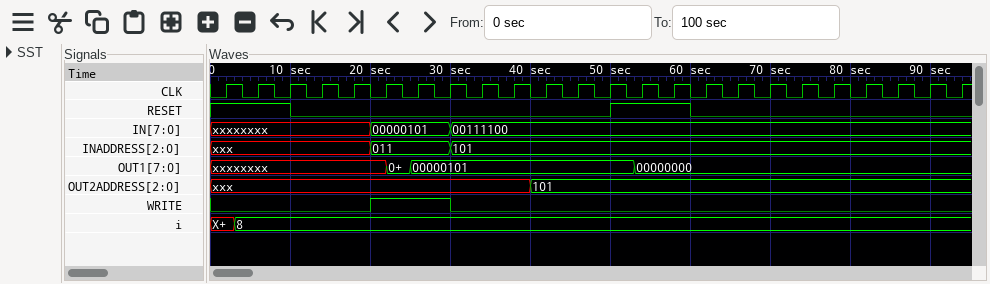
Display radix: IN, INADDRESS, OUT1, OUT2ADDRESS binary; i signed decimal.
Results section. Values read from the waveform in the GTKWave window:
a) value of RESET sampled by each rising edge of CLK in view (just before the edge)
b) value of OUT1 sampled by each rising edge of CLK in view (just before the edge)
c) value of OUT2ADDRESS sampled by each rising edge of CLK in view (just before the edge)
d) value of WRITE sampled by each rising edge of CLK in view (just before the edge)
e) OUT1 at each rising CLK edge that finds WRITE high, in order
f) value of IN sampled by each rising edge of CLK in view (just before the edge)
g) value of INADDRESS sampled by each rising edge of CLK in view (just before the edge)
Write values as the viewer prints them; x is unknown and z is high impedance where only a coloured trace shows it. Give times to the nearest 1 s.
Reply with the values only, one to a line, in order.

1 1 1 0 0 0 0 0 0 0 0 0 0 1 1 0 0 0 0 0 0 0 0 0
xxxxxxxx, xxxxxxxx, xxxxxxxx, xxxxxxxx, xxxxxxxx, xxxxxxxx, 00000101, 00000101, 00000101, 00000101, 00000101, 00000101, 00000101, 00000000, 00000000, 00000000, 00000000, 00000000, 00000000, 00000000, 00000000, 00000000, 00000000, 00000000
xxx, xxx, xxx, xxx, xxx, xxx, xxx, xxx, xxx, xxx, 101, 101, 101, 101, 101, 101, 101, 101, 101, 101, 101, 101, 101, 101
0 0 0 0 0 1 1 1 0 0 0 0 0 0 0 0 0 0 0 0 0 0 0 0
xxxxxxxx, 00000101, 00000101
xxxxxxxx, xxxxxxxx, xxxxxxxx, xxxxxxxx, xxxxxxxx, 00000101, 00000101, 00000101, 00111100, 00111100, 00111100, 00111100, 00111100, 00111100, 00111100, 00111100, 00111100, 00111100, 00111100, 00111100, 00111100, 00111100, 00111100, 00111100
xxx, xxx, xxx, xxx, xxx, 011, 011, 011, 101, 101, 101, 101, 101, 101, 101, 101, 101, 101, 101, 101, 101, 101, 101, 101
